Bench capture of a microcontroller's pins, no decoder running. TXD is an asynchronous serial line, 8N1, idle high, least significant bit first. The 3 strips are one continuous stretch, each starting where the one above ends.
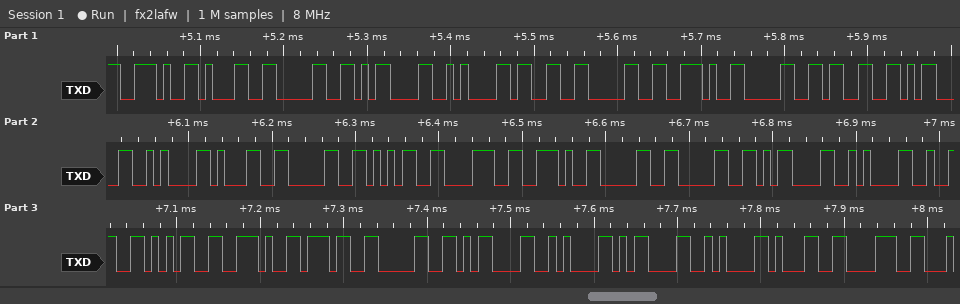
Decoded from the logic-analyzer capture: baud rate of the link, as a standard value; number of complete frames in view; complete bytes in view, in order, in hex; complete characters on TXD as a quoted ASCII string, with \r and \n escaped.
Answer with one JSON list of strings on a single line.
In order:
["115200 baud", "32", "2E 31 30 0D 0A 33 30 2E 30 33 0D 0A 31 30 35 38 2E 30 30 0D 0A 32 35 2E 37 30 0D 0A 0D 0A 31 38", "\".10\\r\\n30.03\\r\\n1058.00\\r\\n25.70\\r\\n\\r\\n18\""]
